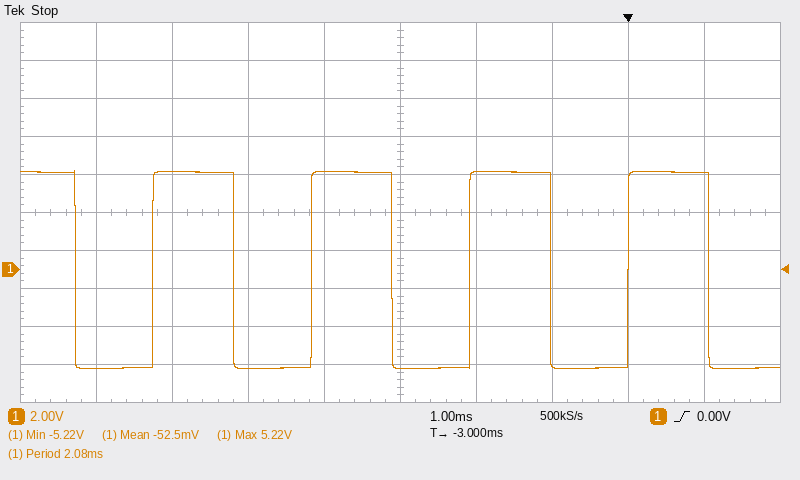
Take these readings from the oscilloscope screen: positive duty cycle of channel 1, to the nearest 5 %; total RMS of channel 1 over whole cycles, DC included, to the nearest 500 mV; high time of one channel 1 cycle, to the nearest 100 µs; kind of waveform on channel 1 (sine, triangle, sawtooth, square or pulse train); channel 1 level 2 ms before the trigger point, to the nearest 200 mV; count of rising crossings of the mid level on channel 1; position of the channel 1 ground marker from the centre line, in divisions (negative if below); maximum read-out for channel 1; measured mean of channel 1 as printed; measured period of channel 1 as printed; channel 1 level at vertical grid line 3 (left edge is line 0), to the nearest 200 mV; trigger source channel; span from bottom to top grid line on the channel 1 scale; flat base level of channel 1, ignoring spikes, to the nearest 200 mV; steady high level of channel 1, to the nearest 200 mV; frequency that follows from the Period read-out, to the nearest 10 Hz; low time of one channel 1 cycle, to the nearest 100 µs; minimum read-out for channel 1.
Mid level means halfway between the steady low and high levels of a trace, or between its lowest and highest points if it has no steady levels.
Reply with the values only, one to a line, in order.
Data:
50 %
5.0 V
1.1 ms
square
5.2 V
4
-1.5 div
5.22 V
-52.5 mV
2.08 ms
-5.2 V
channel 1
20 V
-5.2 V
5.2 V
480 Hz
1.0 ms
-5.22 V
